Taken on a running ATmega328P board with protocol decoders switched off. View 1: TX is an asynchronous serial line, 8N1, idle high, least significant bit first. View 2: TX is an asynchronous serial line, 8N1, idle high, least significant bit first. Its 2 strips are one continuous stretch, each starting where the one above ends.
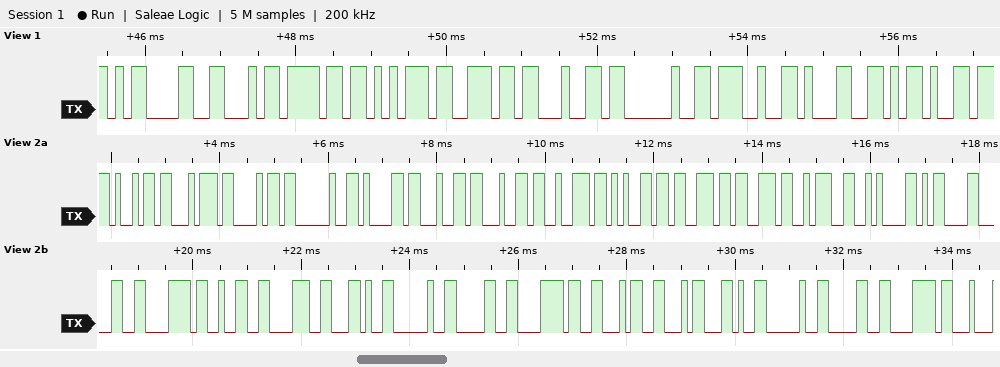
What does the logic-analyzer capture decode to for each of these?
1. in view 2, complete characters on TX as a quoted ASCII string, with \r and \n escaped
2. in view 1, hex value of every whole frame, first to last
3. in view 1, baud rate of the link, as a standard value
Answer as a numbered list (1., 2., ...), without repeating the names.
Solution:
1. "ith address:\n\r0x28, 0xFF, 0x"
2. 0x0D 0x46 0x6F 0x75 0x6E 0x64 0x20 0x27 0x31 0x2D
3. 9600 baud
